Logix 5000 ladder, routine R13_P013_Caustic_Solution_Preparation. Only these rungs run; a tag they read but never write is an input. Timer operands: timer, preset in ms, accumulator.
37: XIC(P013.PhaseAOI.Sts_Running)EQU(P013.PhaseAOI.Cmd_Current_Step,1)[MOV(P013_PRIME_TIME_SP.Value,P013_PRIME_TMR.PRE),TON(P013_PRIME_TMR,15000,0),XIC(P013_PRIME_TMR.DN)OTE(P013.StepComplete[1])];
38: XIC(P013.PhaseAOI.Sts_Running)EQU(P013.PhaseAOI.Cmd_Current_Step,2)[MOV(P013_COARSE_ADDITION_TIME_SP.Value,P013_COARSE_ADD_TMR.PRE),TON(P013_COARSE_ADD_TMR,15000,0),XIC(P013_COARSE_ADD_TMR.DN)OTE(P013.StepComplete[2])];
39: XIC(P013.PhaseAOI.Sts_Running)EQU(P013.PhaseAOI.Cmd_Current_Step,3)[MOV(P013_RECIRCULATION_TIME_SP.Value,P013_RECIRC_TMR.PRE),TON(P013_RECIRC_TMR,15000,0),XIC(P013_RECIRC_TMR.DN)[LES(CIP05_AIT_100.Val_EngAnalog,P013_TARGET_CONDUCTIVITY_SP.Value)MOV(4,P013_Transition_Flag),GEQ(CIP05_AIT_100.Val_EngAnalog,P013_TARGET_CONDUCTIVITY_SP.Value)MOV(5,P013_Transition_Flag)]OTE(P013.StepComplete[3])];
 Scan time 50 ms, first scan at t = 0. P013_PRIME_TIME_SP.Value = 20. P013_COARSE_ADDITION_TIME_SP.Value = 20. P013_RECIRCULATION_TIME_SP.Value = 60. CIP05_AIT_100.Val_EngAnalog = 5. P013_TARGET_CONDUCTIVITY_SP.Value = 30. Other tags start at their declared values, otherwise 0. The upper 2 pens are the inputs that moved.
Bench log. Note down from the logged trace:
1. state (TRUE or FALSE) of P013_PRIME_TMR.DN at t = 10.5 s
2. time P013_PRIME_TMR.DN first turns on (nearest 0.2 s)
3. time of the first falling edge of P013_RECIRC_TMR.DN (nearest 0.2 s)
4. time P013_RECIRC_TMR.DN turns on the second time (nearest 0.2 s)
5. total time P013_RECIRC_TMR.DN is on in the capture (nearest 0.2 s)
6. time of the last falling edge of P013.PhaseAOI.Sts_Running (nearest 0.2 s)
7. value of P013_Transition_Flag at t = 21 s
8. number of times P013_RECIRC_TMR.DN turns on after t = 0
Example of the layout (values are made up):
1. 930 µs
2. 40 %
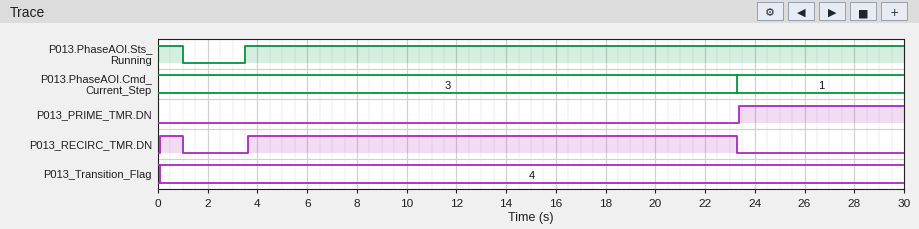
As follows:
1. FALSE
2. 23.4 s
3. 1.0 s
4. 3.6 s
5. 20.6 s
6. 1.0 s
7. 4
8. 2
